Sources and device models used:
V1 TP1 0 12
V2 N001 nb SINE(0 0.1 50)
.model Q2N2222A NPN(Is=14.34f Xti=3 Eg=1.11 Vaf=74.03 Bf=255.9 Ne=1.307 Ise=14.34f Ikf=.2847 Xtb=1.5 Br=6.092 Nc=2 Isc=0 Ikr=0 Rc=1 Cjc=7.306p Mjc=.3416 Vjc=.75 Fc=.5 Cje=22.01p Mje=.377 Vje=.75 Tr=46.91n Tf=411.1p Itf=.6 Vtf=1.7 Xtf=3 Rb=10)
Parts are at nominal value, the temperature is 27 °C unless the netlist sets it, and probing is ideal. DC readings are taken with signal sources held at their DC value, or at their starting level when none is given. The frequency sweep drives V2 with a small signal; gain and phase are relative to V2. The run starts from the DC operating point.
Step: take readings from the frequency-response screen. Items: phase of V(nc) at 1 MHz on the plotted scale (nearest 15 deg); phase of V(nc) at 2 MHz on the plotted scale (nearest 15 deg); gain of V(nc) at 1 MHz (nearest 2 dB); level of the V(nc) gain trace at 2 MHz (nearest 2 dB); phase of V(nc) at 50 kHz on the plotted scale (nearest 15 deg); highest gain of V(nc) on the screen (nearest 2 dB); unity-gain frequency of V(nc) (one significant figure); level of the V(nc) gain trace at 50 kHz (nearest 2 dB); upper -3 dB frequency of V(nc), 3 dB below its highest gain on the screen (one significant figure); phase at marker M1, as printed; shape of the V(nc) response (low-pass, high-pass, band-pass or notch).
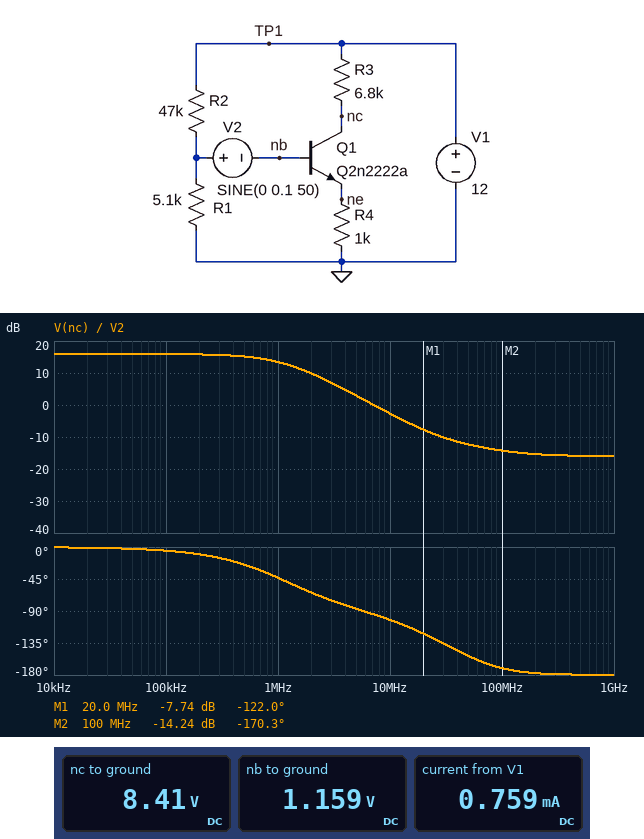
-45 deg
-60 deg
14 dB
10 dB
0 deg
16 dB
7 MHz
16 dB
1 MHz
-122.0 deg
low-pass
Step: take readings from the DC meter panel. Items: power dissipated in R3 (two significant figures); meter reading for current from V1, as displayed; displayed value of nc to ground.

1.9 mW
0.759 mA
8.41 V
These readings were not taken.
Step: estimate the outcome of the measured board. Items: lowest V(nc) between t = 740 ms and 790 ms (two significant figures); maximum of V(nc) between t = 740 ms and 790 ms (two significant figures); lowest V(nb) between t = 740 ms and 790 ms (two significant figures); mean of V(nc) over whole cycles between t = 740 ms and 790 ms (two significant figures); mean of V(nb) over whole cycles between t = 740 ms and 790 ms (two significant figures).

7.8 V
9.0 V
1.1 V
8.4 V
1.2 V
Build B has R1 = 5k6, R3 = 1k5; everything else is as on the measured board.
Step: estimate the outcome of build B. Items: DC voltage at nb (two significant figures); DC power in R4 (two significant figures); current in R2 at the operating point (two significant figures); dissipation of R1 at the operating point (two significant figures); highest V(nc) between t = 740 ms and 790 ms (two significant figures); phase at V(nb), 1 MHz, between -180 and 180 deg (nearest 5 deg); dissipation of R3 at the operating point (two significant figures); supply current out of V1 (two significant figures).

1.3 V
390 µW
230 µA
280 µW
11 V
165 deg
580 µW
850 µA
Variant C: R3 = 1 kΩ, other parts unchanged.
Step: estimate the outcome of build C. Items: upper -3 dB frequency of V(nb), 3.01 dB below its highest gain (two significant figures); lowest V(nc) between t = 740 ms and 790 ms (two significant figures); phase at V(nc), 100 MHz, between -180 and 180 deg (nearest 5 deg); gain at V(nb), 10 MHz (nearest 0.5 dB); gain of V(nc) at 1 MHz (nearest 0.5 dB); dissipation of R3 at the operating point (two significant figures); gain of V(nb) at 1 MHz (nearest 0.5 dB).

4.2 MHz
11 V
-160 deg
-8.5 dB
-1.0 dB
280 µW
-0.5 dB
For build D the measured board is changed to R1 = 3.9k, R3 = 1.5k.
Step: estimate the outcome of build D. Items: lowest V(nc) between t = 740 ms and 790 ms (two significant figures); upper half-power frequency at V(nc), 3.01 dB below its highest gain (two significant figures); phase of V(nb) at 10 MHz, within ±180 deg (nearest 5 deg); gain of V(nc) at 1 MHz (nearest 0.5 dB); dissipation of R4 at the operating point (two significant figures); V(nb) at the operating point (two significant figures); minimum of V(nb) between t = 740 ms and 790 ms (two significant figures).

11 V
4.0 MHz
130 deg
2.5 dB
91 µW
910 mV
810 mV
